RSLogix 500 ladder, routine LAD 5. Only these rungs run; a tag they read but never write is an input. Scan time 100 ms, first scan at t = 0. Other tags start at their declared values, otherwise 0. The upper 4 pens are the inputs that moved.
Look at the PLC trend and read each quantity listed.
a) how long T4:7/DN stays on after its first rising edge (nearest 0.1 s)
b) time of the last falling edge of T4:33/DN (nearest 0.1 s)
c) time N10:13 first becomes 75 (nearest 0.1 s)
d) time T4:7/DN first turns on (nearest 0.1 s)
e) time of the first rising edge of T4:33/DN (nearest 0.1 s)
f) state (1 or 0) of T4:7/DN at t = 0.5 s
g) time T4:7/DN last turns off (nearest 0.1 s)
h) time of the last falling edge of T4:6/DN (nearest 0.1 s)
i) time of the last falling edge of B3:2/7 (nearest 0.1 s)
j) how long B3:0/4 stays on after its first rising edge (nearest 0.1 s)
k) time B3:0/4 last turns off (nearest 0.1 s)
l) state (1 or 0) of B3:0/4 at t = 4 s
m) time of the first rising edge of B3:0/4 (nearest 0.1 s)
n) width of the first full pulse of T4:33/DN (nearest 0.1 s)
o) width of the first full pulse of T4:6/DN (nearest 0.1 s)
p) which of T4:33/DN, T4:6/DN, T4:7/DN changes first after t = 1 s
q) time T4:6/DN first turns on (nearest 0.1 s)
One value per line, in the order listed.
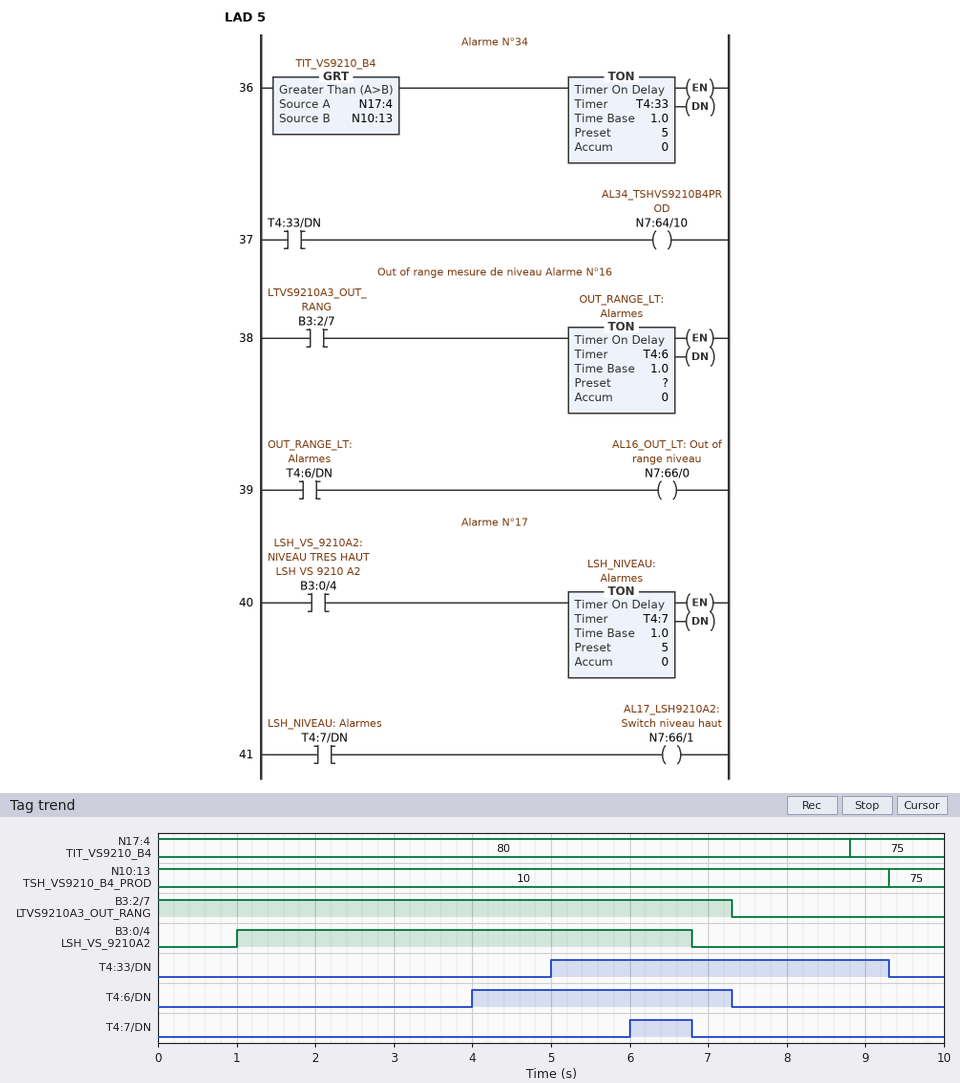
0.8 s
9.3 s
9.3 s
6.0 s
5.0 s
0
6.8 s
7.3 s
7.3 s
5.8 s
6.8 s
1
1.0 s
4.3 s
3.3 s
T4:6/DN
4.0 s
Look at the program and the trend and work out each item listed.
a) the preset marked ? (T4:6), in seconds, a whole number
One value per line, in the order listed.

4 s
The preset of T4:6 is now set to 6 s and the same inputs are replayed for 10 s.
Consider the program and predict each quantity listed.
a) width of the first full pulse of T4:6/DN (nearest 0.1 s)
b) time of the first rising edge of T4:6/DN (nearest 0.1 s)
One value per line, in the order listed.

1.3 s
6.0 s
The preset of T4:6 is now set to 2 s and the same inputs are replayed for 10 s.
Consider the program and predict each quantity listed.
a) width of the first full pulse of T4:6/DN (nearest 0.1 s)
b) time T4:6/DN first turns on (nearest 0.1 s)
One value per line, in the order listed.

5.3 s
2.0 s
